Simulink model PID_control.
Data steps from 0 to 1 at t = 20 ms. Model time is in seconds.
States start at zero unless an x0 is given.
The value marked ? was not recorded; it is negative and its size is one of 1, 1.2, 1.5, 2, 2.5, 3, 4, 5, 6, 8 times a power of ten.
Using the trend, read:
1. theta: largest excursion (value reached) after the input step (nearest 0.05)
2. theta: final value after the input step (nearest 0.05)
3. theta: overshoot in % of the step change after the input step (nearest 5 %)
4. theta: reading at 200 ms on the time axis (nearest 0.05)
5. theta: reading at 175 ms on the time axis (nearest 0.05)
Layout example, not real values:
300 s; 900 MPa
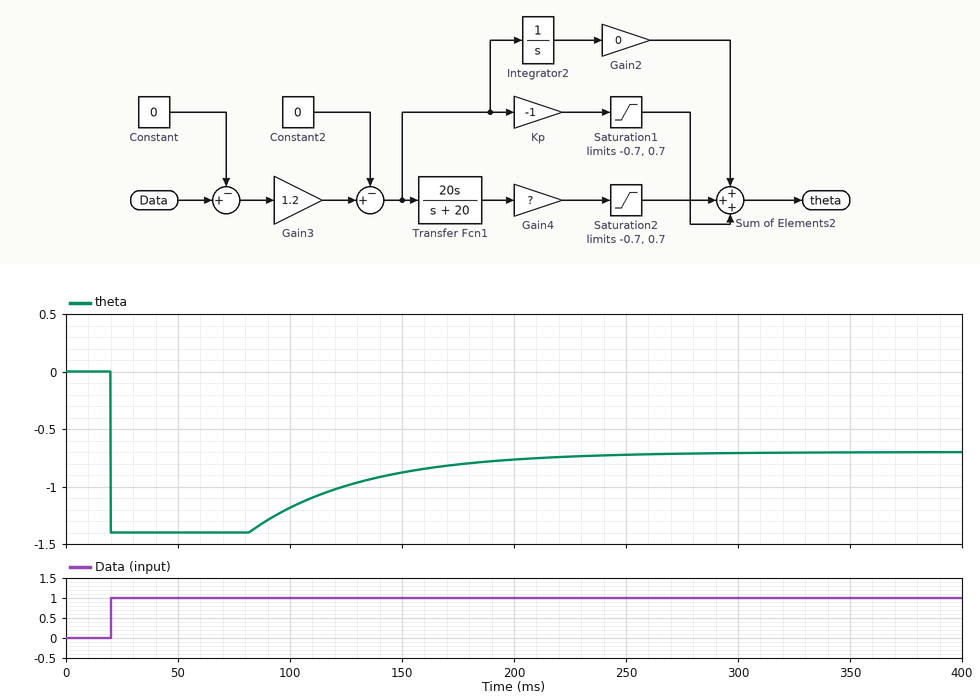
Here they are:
-1.40; -0.70; 100 %; -0.75; -0.80
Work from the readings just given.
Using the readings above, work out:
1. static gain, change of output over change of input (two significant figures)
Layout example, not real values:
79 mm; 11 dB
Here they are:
-0.70
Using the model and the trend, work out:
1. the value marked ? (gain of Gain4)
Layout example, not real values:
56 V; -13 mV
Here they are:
-0.1
